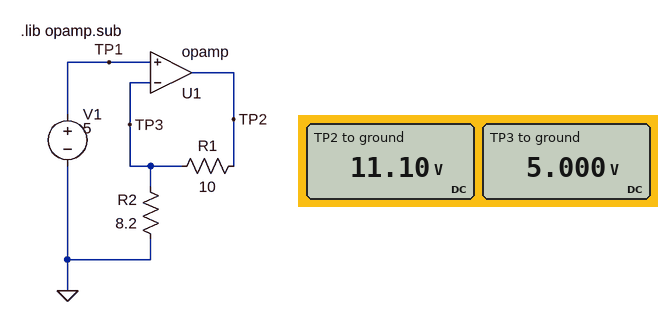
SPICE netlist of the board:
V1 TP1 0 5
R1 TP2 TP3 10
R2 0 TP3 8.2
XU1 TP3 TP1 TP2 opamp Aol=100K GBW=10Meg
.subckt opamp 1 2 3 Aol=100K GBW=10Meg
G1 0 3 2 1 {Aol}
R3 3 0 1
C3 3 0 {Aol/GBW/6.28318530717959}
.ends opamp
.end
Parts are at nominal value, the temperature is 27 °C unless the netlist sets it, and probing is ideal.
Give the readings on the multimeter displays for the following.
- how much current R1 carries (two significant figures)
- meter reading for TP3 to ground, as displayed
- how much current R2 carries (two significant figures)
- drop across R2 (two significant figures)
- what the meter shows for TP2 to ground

610 mA
5.000 V
610 mA
5.0 V
11.10 V
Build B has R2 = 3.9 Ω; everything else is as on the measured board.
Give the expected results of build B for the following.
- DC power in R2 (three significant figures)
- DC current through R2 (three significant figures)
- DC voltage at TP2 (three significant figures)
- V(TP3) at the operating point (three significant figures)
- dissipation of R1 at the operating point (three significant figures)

6.41 W
1.28 A
17.8 V
5.00 V
16.4 W
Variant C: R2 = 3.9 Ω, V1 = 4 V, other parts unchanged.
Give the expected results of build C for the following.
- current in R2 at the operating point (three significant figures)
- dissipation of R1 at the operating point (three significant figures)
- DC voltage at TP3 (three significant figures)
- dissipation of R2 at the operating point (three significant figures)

1.03 A
10.5 W
4.00 V
4.10 W
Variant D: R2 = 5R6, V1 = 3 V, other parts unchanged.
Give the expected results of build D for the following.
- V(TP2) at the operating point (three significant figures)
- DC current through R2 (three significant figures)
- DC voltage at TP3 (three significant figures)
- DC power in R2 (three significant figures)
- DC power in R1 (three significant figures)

8.36 V
536 mA
3.00 V
1.61 W
2.87 W
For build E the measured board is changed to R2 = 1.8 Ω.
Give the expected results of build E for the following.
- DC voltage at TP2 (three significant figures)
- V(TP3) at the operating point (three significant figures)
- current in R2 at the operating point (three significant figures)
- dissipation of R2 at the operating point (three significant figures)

32.8 V
5.00 V
2.78 A
13.9 W
